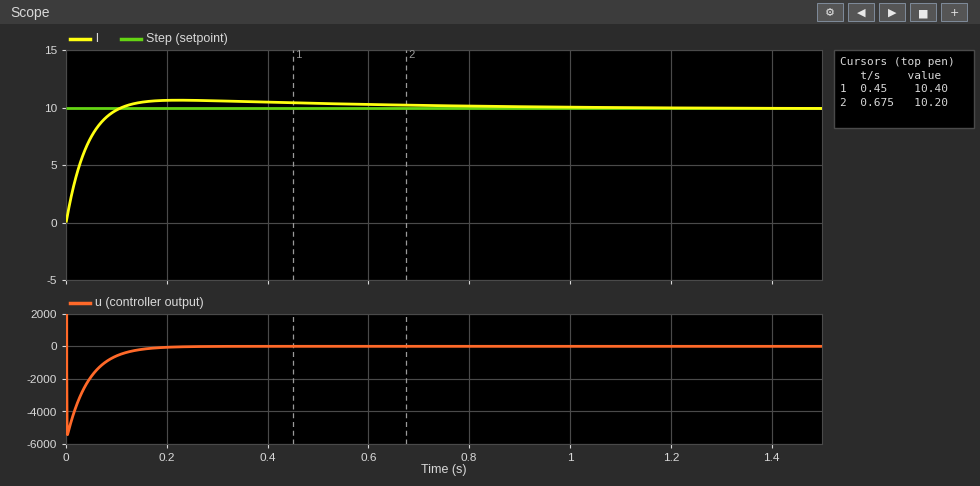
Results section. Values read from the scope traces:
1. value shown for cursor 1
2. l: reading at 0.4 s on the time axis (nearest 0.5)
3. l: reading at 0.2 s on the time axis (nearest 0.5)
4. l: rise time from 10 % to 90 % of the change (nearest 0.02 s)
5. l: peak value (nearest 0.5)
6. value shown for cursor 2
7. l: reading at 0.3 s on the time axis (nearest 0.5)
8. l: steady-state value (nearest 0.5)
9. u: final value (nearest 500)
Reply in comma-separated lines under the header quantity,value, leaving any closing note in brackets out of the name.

quantity,value
value shown for cursor 1,10.40
l: reading at 0.4 s on the time axis,10.5
l: reading at 0.2 s on the time axis,10.5
l: rise time from 10 % to 90 % of the change,0.08 s
l: peak value,10.5
value shown for cursor 2,10.20
l: reading at 0.3 s on the time axis,10.5
l: steady-state value,10.0
u: final value,0
